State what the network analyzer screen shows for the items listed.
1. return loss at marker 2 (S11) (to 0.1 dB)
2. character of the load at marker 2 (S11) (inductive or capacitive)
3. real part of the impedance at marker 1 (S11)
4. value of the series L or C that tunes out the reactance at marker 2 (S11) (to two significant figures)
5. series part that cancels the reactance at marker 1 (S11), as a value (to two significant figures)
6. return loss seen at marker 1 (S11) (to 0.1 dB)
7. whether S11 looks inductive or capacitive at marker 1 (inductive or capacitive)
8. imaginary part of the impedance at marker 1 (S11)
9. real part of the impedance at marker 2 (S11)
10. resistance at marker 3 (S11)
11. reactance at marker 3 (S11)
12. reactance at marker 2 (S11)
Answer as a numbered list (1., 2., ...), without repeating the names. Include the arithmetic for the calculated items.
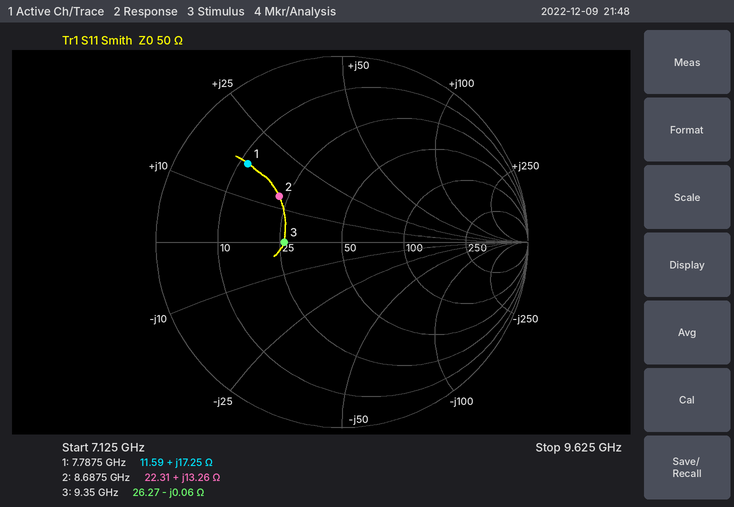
1. 7.6 dB
2. inductive
3. 11.59 Ω
4. C = 1/(2π × 8.6875 GHz × 13.26 Ω) ≈ 1.4 pF
5. C = 1/(2π × 7.7875 GHz × 17.25 Ω) ≈ 1.2 pF
6. 3.6 dB
7. inductive
8. +17.25 Ω
9. 22.31 Ω
10. 26.27 Ω
11. -0.06 Ω
12. +13.26 Ω
